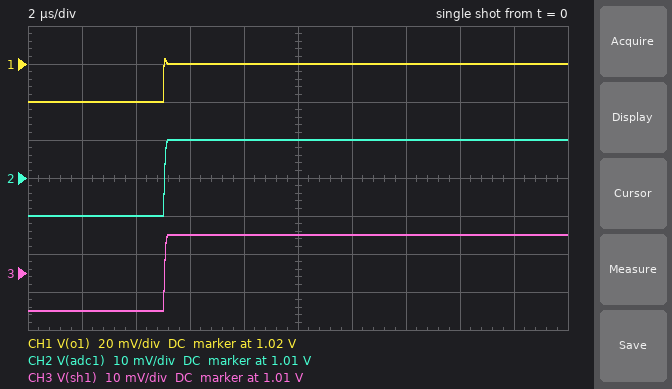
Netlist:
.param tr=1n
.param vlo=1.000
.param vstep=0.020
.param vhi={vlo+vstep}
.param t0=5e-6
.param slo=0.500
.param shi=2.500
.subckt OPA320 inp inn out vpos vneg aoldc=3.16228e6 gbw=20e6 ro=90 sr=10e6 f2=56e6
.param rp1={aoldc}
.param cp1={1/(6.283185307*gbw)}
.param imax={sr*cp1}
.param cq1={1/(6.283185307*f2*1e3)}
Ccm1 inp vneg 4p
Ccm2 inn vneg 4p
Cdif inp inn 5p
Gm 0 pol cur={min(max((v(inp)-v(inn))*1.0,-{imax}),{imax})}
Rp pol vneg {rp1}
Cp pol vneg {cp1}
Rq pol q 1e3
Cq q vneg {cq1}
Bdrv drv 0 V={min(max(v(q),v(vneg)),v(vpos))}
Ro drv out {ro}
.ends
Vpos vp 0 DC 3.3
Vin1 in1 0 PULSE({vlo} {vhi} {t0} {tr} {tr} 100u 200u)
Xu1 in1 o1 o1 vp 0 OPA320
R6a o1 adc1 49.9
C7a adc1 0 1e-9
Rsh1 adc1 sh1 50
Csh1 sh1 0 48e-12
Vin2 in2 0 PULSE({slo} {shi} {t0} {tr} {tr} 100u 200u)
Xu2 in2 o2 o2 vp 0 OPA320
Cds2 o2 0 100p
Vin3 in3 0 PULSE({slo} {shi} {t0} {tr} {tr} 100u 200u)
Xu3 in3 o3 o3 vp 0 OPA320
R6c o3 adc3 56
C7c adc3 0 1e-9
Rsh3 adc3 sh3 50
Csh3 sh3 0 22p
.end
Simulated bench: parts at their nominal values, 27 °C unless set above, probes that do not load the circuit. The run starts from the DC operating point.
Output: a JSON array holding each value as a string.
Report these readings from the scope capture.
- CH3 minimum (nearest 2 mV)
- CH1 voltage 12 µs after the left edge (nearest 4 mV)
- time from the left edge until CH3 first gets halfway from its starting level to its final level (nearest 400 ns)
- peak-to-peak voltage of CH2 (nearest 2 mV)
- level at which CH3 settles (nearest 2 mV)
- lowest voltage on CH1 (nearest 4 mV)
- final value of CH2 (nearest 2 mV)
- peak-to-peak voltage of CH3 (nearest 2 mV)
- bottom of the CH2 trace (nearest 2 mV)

["1.000 V", "1.020 V", "5.2 µs", "20 mV", "1.020 V", "1.000 V", "1.020 V", "20 mV", "1.000 V"]
